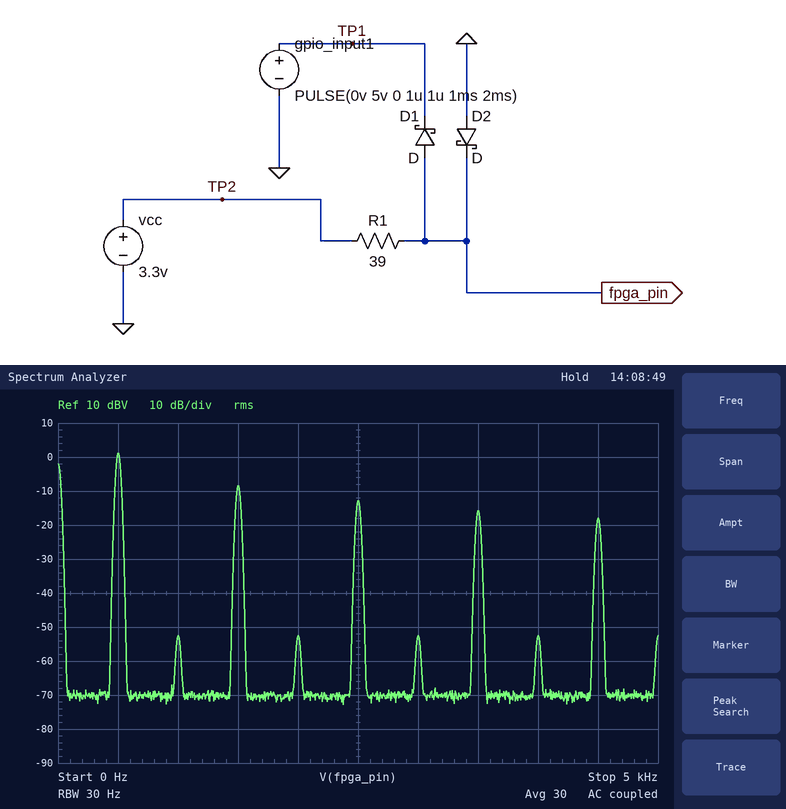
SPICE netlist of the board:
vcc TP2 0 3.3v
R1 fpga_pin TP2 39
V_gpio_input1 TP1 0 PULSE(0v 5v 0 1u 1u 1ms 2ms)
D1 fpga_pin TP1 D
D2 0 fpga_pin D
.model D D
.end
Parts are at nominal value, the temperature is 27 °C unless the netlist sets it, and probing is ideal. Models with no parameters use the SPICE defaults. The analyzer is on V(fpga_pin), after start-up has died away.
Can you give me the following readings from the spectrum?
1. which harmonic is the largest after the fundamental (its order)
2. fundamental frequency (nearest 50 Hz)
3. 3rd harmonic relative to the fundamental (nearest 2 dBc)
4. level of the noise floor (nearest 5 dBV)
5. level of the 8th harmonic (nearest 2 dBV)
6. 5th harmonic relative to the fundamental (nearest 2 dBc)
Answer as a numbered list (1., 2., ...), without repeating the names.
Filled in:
1. 3
2. 500 Hz
3. -10 dBc
4. -70 dBV
5. -52 dBV
6. -14 dBc
